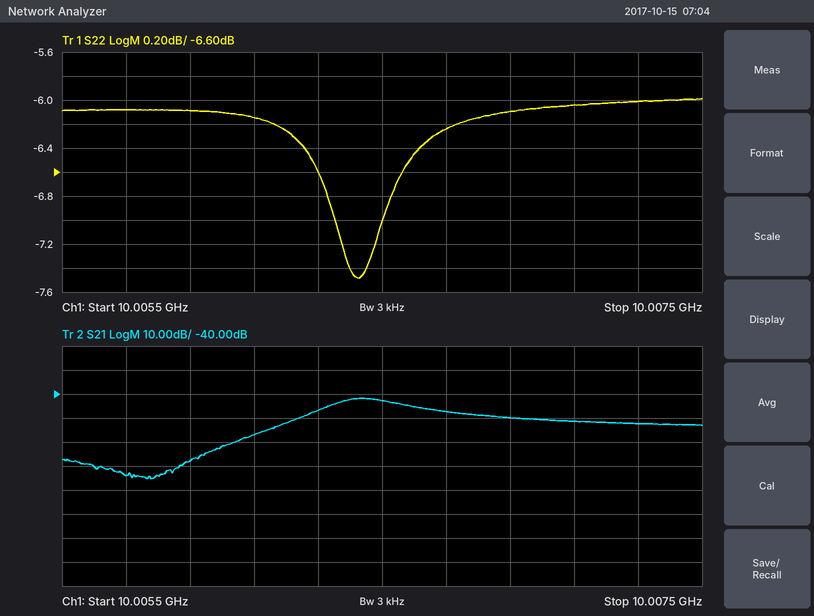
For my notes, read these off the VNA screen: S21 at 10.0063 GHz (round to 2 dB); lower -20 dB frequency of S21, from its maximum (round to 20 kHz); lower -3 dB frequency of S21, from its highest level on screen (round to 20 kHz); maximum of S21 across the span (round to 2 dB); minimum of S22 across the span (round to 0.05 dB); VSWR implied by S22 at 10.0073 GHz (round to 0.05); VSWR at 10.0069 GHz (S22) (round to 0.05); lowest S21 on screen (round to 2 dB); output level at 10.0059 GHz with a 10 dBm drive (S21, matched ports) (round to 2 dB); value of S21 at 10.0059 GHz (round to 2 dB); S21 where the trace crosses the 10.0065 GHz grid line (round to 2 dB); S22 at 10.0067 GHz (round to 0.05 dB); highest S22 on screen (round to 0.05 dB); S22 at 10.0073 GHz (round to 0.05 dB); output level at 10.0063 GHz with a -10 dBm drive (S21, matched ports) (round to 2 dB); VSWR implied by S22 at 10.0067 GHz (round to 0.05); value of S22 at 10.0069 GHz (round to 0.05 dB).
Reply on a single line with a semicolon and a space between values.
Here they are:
-46 dB; 10.00600 GHz; 10.00634 GHz; -42 dB; -7.50 dB; 3.00; 2.95; -76 dB; -58 dBm; -68 dB; -42 dB; -6.25 dB; -6.00 dB; -6.00 dB; -56 dBm; 2.90; -6.10 dB
